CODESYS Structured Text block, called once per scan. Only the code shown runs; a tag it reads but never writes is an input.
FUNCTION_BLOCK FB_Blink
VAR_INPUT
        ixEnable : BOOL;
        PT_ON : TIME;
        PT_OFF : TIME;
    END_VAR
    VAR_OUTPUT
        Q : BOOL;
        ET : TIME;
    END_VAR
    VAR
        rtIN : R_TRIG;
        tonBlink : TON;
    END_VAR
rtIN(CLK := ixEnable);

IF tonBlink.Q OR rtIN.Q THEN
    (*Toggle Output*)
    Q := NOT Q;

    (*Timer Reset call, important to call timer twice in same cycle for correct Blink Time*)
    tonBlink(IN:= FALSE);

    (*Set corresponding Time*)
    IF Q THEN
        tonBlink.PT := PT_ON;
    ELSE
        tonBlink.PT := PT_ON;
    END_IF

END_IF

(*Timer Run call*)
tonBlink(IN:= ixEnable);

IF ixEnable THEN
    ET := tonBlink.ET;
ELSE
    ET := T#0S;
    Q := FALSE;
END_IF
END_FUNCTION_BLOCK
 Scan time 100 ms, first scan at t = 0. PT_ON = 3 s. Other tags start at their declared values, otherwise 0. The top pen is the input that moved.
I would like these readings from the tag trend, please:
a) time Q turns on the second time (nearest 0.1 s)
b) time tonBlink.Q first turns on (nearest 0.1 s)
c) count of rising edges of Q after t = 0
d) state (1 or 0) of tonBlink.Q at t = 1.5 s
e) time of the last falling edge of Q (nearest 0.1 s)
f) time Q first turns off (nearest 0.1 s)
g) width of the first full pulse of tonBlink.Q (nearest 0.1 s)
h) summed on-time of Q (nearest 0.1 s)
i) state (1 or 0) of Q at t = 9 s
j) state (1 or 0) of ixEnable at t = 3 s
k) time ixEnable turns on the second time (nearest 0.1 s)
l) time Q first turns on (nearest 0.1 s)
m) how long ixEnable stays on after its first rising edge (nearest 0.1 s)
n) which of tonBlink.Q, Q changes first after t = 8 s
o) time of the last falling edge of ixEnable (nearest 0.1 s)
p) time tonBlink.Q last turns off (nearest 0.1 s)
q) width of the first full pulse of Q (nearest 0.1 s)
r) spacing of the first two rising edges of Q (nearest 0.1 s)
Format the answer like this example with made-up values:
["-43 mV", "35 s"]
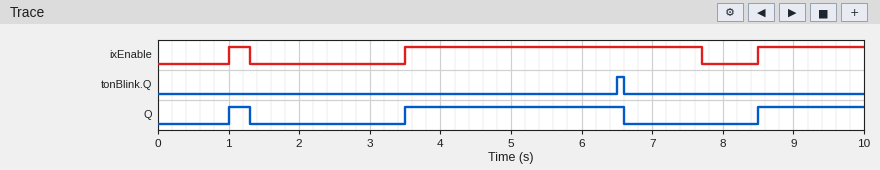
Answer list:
["3.5 s", "6.5 s", "3", "0", "6.6 s", "1.3 s", "0.1 s", "4.9 s", "1", "0", "3.5 s", "1.0 s", "0.3 s", "Q", "7.7 s", "6.6 s", "0.3 s", "2.5 s"]
